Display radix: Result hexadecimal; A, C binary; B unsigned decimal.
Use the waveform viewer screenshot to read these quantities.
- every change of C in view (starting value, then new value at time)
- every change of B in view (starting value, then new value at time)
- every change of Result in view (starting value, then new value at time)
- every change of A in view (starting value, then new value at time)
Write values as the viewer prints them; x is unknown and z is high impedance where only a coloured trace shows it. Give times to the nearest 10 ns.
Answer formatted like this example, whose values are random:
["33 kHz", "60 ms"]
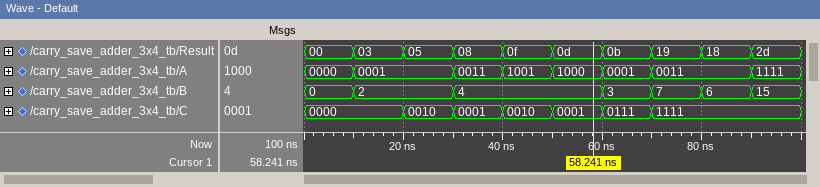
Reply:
["0000, 0010 at 20 ns, 0001 at 30 ns, 0010 at 40 ns, 0001 at 50 ns, 0111 at 60 ns, 1111 at 70 ns", "0, 2 at 10 ns, 4 at 30 ns, 3 at 60 ns, 7 at 70 ns, 6 at 80 ns, 15 at 90 ns", "00, 03 at 10 ns, 05 at 20 ns, 08 at 30 ns, 0f at 40 ns, 0d at 50 ns, 0b at 60 ns, 19 at 70 ns, 18 at 80 ns, 2d at 90 ns", "0000, 0001 at 10 ns, 0011 at 30 ns, 1001 at 40 ns, 1000 at 50 ns, 0001 at 60 ns, 0011 at 70 ns, 1111 at 90 ns"]
